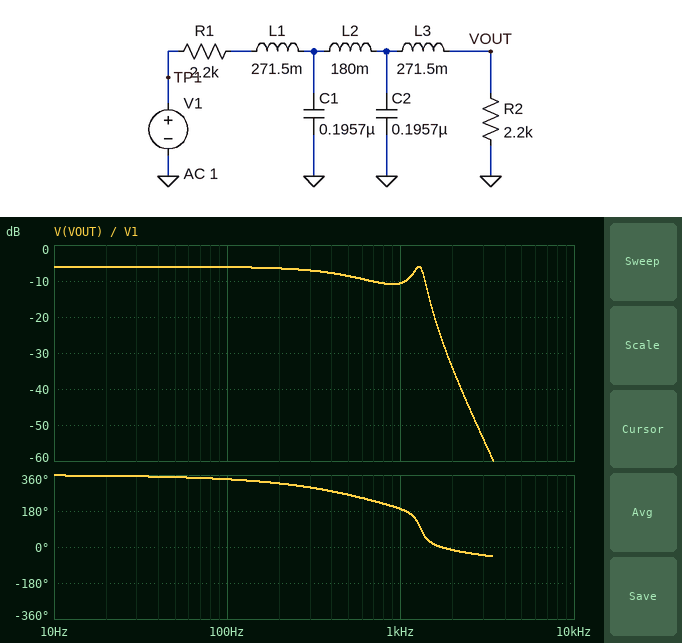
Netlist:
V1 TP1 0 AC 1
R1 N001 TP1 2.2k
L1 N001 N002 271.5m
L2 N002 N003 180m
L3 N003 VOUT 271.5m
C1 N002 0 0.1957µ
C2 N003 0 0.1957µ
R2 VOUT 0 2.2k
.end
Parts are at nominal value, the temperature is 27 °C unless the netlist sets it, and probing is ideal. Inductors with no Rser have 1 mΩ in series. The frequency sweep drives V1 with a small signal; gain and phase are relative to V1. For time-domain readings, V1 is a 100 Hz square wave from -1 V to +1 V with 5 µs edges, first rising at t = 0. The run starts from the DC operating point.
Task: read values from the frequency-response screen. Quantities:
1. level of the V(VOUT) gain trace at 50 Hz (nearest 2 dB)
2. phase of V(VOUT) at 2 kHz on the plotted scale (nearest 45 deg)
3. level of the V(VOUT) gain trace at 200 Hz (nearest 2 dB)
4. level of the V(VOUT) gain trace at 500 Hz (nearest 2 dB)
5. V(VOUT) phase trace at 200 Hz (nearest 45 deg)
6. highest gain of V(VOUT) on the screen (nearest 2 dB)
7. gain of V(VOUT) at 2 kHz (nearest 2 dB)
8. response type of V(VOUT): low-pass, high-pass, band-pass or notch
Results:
-6 dB
0 deg
-6 dB
-8 dB
315 deg
-6 dB
-34 dB
low-pass
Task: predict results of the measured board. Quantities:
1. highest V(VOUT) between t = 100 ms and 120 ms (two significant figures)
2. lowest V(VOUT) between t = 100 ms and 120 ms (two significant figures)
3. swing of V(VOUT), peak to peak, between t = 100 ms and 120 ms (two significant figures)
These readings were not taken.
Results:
560 mV
-560 mV
1.1 V
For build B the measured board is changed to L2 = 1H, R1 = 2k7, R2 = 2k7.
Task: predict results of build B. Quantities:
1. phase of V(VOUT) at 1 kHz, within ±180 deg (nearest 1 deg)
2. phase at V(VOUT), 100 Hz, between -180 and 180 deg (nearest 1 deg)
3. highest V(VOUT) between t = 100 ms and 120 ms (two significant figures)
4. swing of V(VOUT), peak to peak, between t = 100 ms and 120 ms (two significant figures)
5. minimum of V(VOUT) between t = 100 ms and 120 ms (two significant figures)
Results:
59 deg
-29 deg
610 mV
1.2 V
-610 mV
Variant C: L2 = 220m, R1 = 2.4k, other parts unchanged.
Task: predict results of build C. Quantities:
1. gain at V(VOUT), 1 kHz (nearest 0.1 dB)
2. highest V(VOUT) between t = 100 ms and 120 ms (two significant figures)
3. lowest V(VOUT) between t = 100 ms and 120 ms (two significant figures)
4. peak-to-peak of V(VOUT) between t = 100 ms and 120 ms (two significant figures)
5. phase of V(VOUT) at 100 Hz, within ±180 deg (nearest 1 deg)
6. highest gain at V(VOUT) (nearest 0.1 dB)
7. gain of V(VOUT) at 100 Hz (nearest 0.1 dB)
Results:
-8.9 dB
530 mV
-530 mV
1.1 V
-22 deg
-6.4 dB
-6.5 dB
